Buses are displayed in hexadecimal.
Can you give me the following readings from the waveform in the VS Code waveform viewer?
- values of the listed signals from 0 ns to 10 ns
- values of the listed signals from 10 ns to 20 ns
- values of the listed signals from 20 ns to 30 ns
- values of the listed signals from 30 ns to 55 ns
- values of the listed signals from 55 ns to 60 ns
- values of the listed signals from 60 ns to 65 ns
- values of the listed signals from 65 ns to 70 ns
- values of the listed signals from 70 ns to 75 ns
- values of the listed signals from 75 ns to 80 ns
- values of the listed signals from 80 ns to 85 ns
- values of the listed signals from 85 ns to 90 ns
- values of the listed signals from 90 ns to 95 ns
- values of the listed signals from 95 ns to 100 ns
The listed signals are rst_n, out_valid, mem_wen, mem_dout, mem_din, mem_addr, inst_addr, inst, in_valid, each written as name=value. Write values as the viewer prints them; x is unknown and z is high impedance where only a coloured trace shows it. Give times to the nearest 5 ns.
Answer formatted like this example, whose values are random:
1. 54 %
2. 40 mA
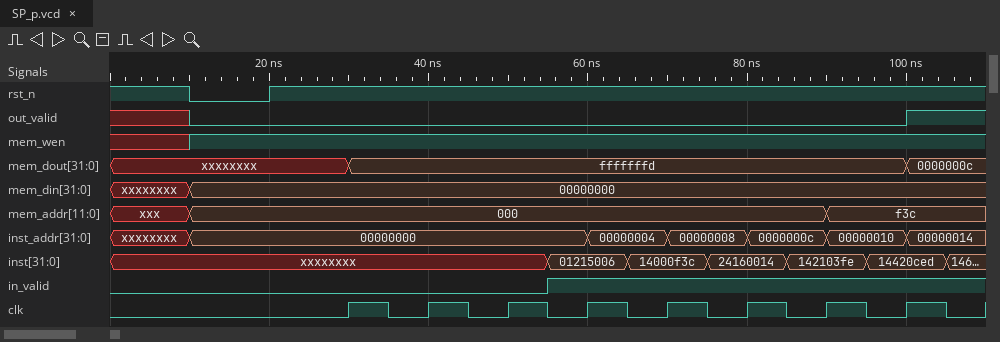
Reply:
1. rst_n=1, out_valid=x, mem_wen=x, mem_dout=xxxxxxxx, mem_din=xxxxxxxx, mem_addr=xxx, inst_addr=xxxxxxxx, inst=xxxxxxxx, in_valid=0
2. rst_n=0, out_valid=0, mem_wen=1, mem_dout=xxxxxxxx, mem_din=00000000, mem_addr=000, inst_addr=00000000, inst=xxxxxxxx, in_valid=0
3. rst_n=1, out_valid=0, mem_wen=1, mem_dout=xxxxxxxx, mem_din=00000000, mem_addr=000, inst_addr=00000000, inst=xxxxxxxx, in_valid=0
4. rst_n=1, out_valid=0, mem_wen=1, mem_dout=fffffffd, mem_din=00000000, mem_addr=000, inst_addr=00000000, inst=xxxxxxxx, in_valid=0
5. rst_n=1, out_valid=0, mem_wen=1, mem_dout=fffffffd, mem_din=00000000, mem_addr=000, inst_addr=00000000, inst=01215006, in_valid=1
6. rst_n=1, out_valid=0, mem_wen=1, mem_dout=fffffffd, mem_din=00000000, mem_addr=000, inst_addr=00000004, inst=01215006, in_valid=1
7. rst_n=1, out_valid=0, mem_wen=1, mem_dout=fffffffd, mem_din=00000000, mem_addr=000, inst_addr=00000004, inst=14000f3c, in_valid=1
8. rst_n=1, out_valid=0, mem_wen=1, mem_dout=fffffffd, mem_din=00000000, mem_addr=000, inst_addr=00000008, inst=14000f3c, in_valid=1
9. rst_n=1, out_valid=0, mem_wen=1, mem_dout=fffffffd, mem_din=00000000, mem_addr=000, inst_addr=00000008, inst=24160014, in_valid=1
10. rst_n=1, out_valid=0, mem_wen=1, mem_dout=fffffffd, mem_din=00000000, mem_addr=000, inst_addr=0000000c, inst=24160014, in_valid=1
11. rst_n=1, out_valid=0, mem_wen=1, mem_dout=fffffffd, mem_din=00000000, mem_addr=000, inst_addr=0000000c, inst=142103fe, in_valid=1
12. rst_n=1, out_valid=0, mem_wen=1, mem_dout=fffffffd, mem_din=00000000, mem_addr=f3c, inst_addr=00000010, inst=142103fe, in_valid=1
13. rst_n=1, out_valid=0, mem_wen=1, mem_dout=fffffffd, mem_din=00000000, mem_addr=f3c, inst_addr=00000010, inst=14420ced, in_valid=1
